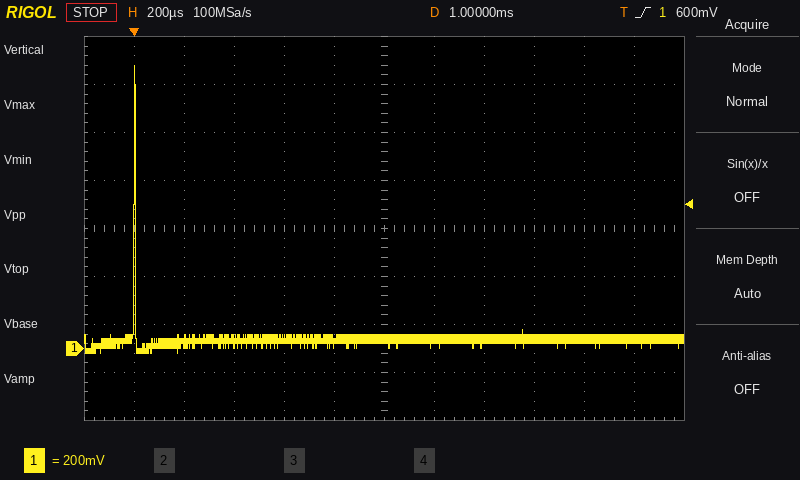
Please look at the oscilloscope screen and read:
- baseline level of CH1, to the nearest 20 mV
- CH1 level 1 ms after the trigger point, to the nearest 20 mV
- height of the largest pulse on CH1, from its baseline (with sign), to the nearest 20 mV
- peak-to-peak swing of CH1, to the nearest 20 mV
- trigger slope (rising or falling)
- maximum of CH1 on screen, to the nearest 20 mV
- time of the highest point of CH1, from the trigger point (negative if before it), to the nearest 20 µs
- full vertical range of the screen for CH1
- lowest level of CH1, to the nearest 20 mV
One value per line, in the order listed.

40 mV
40 mV
+1.14 V
1.20 V
rising
1.18 V
0 µs
1.6 V
-20 mV
